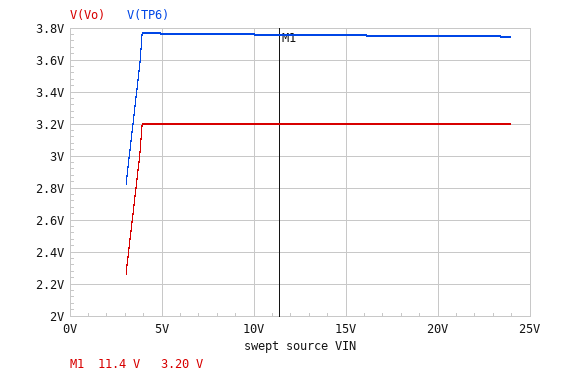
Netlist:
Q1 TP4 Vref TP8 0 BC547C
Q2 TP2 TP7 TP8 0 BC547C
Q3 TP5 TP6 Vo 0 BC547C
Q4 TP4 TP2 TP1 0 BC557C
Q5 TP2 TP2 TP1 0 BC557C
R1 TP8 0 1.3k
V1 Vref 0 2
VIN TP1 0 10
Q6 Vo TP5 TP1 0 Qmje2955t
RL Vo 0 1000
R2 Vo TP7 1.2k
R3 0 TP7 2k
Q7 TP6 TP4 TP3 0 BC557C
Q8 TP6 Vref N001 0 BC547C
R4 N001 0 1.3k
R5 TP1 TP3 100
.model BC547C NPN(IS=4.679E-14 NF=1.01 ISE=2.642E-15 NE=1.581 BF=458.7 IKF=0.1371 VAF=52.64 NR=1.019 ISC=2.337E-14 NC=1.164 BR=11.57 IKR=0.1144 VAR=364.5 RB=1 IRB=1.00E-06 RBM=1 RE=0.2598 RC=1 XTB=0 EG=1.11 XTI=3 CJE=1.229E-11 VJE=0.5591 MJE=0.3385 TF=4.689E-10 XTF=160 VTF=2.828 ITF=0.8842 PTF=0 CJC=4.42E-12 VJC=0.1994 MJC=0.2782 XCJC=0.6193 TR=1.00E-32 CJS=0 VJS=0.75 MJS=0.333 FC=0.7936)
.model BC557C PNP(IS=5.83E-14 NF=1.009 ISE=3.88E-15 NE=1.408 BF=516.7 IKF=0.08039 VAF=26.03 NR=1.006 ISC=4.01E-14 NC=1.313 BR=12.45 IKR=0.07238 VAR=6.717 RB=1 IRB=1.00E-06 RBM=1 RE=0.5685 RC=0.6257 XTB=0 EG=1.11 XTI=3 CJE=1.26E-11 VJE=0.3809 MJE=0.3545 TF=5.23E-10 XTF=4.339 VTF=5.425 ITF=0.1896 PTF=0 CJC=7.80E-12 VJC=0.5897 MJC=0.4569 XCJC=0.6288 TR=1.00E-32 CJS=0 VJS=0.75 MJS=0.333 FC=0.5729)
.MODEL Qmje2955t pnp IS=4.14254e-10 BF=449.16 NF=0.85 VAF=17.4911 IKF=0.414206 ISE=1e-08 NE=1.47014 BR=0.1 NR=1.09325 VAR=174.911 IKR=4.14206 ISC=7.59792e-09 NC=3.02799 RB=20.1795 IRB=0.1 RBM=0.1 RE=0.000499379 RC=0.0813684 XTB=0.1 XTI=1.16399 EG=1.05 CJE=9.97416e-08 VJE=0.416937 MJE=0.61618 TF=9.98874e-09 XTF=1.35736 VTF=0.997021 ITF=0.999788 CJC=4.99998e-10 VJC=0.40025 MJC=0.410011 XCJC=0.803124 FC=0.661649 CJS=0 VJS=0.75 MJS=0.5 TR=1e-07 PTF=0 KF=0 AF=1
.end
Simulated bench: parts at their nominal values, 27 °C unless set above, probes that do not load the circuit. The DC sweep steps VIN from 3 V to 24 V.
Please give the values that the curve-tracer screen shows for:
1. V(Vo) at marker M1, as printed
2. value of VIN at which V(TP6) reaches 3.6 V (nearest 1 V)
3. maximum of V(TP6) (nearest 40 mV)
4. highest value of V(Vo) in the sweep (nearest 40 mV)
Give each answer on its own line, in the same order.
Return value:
3.20 V
4 V
3.76 V
3.20 V
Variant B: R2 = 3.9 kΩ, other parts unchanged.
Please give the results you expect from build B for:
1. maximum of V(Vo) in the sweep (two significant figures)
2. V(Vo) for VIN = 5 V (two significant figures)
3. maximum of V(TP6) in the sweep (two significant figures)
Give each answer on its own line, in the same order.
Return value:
5.9 V
4.2 V
6.5 V
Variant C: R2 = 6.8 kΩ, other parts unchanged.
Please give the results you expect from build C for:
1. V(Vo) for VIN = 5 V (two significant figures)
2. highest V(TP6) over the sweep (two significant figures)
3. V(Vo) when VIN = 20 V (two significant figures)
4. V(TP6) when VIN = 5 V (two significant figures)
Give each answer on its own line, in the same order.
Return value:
4.2 V
9.4 V
8.8 V
4.8 V
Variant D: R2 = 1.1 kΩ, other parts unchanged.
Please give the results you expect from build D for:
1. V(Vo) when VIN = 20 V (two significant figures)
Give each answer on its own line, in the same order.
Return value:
3.1 V
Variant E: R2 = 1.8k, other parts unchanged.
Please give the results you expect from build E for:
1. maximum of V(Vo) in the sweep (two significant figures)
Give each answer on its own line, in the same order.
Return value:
3.8 V
